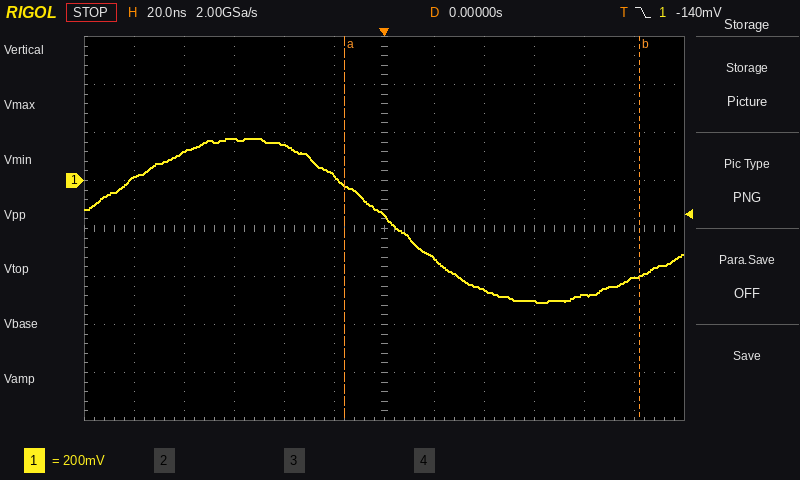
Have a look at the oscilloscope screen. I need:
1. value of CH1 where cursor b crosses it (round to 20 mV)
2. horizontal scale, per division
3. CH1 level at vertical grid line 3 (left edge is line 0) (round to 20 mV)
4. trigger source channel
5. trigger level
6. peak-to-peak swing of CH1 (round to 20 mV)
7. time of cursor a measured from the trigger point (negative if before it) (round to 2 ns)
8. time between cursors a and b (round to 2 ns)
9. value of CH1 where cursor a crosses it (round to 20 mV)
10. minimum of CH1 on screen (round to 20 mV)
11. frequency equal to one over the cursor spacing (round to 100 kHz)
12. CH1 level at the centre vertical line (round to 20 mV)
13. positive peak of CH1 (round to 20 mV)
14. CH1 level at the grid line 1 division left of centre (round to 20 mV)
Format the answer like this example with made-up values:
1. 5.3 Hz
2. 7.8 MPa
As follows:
1. -400 mV
2. 20 ns
3. 180 mV
4. CH1
5. -140 mV
6. 680 mV
7. -16 ns
8. 118 ns
9. -20 mV
10. -500 mV
11. 8.5 MHz
12. -140 mV
13. 180 mV
14. 20 mV
